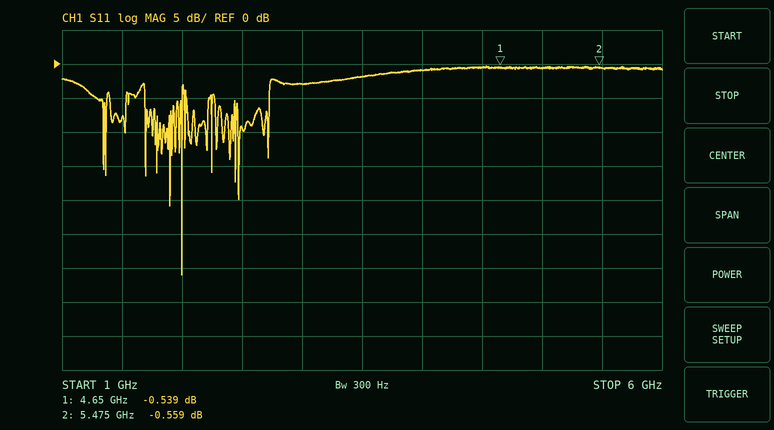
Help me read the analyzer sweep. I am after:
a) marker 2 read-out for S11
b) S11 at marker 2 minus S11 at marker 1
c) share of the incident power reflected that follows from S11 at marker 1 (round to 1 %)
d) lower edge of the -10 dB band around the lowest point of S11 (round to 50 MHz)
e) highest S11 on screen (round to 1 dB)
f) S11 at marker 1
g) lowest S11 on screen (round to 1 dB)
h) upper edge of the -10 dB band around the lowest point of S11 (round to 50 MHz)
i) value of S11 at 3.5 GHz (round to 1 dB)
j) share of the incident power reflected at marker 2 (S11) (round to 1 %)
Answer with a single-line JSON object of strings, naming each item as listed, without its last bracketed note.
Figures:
{"marker 2 read-out for S11": "-0.559 dB", "S11 at marker 2 minus S11 at marker 1": "-0.020 dB", "share of the incident power reflected that follows from S11 at marker 1": "88 %", "lower edge of the -10 dB band around the lowest point of S11": "2.00 GHz", "highest S11 on screen": "0 dB", "S11 at marker 1": "-0.539 dB", "lowest S11 on screen": "-31 dB", "upper edge of the -10 dB band around the lowest point of S11": "2.00 GHz", "value of S11 at 3.5 GHz": "-2 dB", "share of the incident power reflected at marker 2 (S11)": "88 %"}
